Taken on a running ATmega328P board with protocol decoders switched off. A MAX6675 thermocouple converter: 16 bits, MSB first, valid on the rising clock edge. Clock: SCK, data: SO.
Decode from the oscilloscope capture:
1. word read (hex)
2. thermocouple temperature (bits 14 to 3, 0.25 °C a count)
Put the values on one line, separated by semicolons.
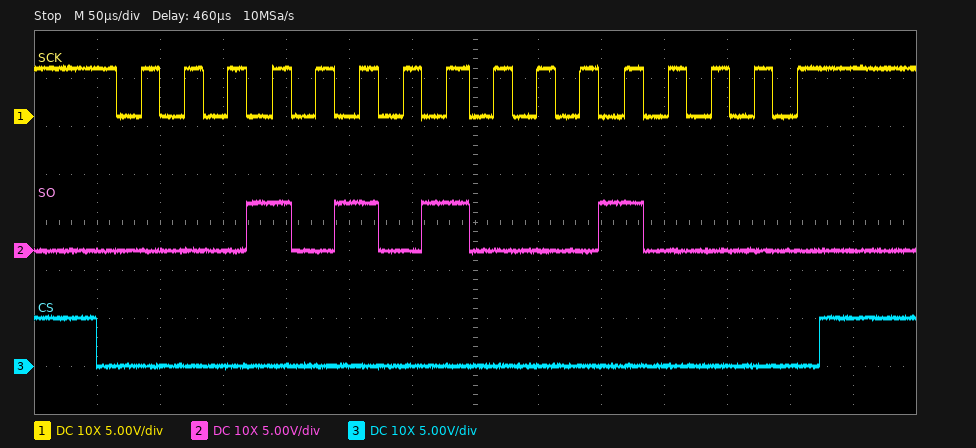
0x1510; 168.50 °C
